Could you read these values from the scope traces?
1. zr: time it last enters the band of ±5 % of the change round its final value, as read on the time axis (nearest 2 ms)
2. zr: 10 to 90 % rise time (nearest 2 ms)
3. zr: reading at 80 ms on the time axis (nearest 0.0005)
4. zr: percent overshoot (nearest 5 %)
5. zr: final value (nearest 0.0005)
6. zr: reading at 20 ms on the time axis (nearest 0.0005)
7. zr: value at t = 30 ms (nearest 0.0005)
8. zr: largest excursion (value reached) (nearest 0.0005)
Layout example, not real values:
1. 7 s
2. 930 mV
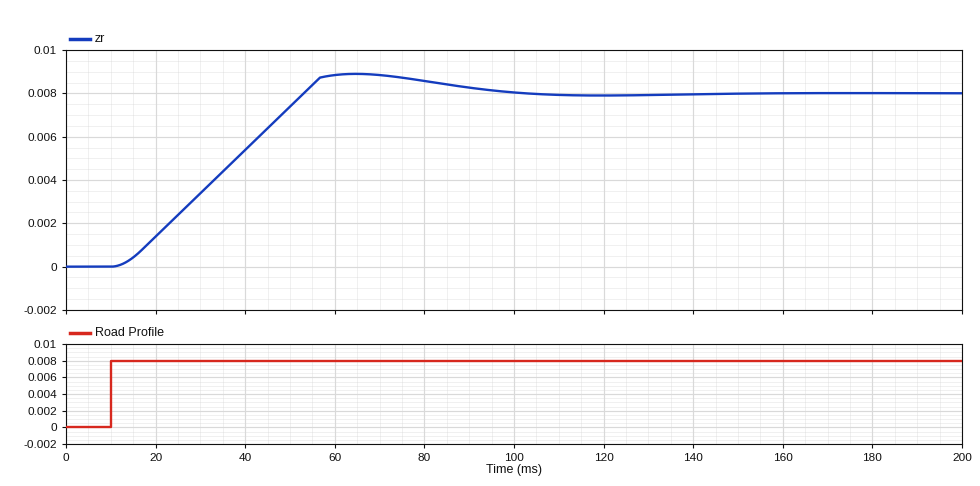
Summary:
1. 86 ms
2. 32 ms
3. 0.0085
4. 10 %
5. 0.0080
6. 0.0015
7. 0.0035
8. 0.0090
